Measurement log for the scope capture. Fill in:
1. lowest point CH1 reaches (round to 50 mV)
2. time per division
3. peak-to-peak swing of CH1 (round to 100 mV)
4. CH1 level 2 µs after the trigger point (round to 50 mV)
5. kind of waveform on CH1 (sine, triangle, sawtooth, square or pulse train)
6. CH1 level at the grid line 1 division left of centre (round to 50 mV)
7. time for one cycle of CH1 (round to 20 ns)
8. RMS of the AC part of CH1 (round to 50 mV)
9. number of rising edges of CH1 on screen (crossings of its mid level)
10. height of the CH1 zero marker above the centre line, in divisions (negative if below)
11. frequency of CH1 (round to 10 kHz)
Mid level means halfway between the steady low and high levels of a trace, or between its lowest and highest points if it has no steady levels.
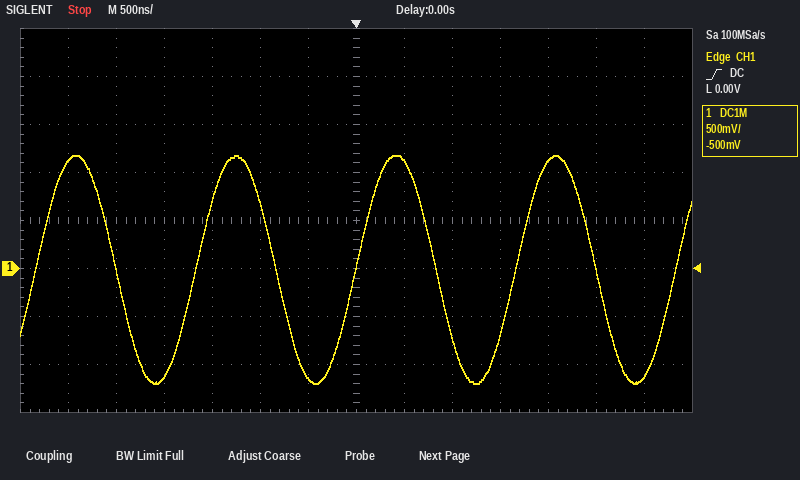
-1.20 V
500 ns
2.40 V
1.10 V
sine
-1.15 V
1.66 µs
850 mV
5
-1.0 div
600 kHz
